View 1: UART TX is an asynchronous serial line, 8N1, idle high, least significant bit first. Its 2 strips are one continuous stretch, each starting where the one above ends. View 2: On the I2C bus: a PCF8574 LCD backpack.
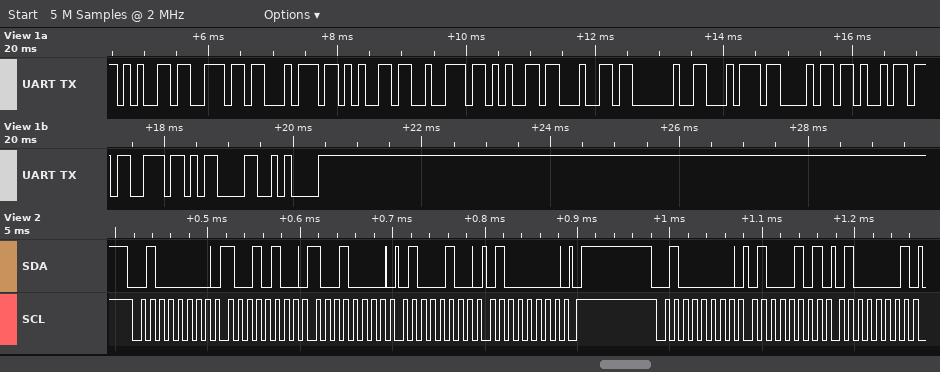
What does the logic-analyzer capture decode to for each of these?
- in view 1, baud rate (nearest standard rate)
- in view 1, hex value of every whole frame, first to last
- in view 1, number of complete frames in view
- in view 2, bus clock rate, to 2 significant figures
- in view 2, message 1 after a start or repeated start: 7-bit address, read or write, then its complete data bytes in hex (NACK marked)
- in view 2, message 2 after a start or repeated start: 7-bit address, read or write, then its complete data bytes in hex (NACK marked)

9600 baud
0x65 0x6E 0x74 0x65 0x72 0x65 0x64 0x20 0x74 0x68 0x69 0x73 0x0D 0x0A
14
100 kHz
0x20 write: 94 90 44 40
0x20 write: 45 41
